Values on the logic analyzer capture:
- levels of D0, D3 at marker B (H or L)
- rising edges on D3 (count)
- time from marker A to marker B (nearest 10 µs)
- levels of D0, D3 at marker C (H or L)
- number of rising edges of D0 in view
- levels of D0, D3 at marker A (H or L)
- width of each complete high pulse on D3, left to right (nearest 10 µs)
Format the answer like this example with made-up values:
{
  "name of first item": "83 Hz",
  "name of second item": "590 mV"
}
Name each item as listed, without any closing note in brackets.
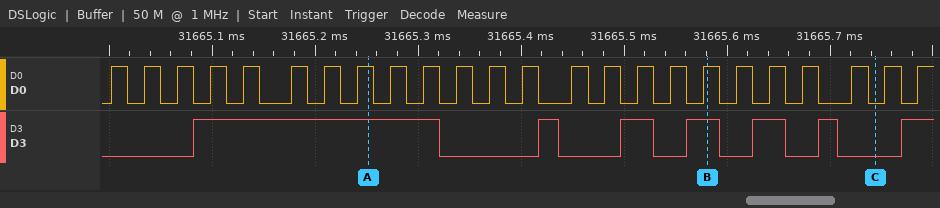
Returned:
{
  "levels of D0, D3 at marker B": "D0=H, D3=H",
  "rising edges on D3": "7",
  "time from marker A to marker B": "330 µs",
  "levels of D0, D3 at marker C": "D0=L, D3=L",
  "number of rising edges of D0 in view": "24",
  "levels of D0, D3 at marker A": "D0=H, D3=H",
  "width of each complete high pulse on D3, left to right": "240 µs, 20 µs, 30 µs, 30 µs, 30 µs, 20 µs"
}
